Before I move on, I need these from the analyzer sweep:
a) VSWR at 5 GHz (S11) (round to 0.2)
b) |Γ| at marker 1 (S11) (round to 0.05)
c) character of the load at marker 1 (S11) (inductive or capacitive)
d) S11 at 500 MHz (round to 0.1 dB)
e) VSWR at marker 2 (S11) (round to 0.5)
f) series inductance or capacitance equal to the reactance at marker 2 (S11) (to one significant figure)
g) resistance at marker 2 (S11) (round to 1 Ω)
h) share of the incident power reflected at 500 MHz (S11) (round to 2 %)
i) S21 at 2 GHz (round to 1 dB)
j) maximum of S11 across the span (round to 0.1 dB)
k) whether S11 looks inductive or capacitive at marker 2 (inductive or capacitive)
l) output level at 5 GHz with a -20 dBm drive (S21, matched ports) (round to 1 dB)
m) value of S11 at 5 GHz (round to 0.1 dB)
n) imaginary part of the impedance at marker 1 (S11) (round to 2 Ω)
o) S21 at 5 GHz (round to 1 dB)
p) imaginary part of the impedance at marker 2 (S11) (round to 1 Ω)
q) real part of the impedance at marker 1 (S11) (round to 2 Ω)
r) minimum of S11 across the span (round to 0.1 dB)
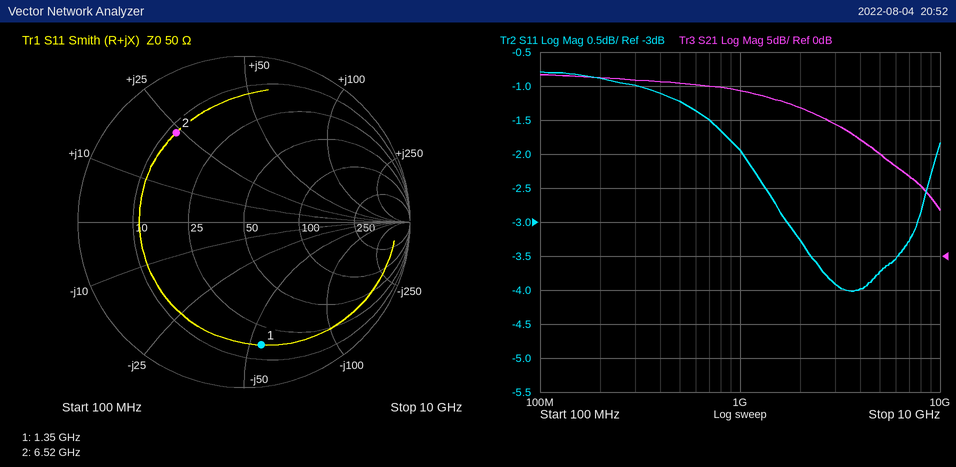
4.8
0.75
capacitive
-1.2 dB
5.0
600 pH
12 Ω
76 %
22 dB
-0.8 dB
inductive
-5 dBm
-3.7 dB
-54 Ω
15 dB
+24 Ω
16 Ω
-4.0 dB
